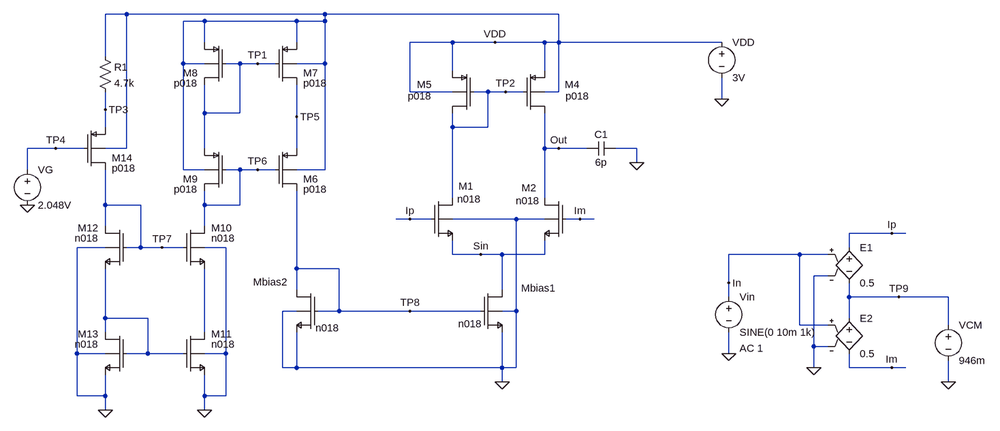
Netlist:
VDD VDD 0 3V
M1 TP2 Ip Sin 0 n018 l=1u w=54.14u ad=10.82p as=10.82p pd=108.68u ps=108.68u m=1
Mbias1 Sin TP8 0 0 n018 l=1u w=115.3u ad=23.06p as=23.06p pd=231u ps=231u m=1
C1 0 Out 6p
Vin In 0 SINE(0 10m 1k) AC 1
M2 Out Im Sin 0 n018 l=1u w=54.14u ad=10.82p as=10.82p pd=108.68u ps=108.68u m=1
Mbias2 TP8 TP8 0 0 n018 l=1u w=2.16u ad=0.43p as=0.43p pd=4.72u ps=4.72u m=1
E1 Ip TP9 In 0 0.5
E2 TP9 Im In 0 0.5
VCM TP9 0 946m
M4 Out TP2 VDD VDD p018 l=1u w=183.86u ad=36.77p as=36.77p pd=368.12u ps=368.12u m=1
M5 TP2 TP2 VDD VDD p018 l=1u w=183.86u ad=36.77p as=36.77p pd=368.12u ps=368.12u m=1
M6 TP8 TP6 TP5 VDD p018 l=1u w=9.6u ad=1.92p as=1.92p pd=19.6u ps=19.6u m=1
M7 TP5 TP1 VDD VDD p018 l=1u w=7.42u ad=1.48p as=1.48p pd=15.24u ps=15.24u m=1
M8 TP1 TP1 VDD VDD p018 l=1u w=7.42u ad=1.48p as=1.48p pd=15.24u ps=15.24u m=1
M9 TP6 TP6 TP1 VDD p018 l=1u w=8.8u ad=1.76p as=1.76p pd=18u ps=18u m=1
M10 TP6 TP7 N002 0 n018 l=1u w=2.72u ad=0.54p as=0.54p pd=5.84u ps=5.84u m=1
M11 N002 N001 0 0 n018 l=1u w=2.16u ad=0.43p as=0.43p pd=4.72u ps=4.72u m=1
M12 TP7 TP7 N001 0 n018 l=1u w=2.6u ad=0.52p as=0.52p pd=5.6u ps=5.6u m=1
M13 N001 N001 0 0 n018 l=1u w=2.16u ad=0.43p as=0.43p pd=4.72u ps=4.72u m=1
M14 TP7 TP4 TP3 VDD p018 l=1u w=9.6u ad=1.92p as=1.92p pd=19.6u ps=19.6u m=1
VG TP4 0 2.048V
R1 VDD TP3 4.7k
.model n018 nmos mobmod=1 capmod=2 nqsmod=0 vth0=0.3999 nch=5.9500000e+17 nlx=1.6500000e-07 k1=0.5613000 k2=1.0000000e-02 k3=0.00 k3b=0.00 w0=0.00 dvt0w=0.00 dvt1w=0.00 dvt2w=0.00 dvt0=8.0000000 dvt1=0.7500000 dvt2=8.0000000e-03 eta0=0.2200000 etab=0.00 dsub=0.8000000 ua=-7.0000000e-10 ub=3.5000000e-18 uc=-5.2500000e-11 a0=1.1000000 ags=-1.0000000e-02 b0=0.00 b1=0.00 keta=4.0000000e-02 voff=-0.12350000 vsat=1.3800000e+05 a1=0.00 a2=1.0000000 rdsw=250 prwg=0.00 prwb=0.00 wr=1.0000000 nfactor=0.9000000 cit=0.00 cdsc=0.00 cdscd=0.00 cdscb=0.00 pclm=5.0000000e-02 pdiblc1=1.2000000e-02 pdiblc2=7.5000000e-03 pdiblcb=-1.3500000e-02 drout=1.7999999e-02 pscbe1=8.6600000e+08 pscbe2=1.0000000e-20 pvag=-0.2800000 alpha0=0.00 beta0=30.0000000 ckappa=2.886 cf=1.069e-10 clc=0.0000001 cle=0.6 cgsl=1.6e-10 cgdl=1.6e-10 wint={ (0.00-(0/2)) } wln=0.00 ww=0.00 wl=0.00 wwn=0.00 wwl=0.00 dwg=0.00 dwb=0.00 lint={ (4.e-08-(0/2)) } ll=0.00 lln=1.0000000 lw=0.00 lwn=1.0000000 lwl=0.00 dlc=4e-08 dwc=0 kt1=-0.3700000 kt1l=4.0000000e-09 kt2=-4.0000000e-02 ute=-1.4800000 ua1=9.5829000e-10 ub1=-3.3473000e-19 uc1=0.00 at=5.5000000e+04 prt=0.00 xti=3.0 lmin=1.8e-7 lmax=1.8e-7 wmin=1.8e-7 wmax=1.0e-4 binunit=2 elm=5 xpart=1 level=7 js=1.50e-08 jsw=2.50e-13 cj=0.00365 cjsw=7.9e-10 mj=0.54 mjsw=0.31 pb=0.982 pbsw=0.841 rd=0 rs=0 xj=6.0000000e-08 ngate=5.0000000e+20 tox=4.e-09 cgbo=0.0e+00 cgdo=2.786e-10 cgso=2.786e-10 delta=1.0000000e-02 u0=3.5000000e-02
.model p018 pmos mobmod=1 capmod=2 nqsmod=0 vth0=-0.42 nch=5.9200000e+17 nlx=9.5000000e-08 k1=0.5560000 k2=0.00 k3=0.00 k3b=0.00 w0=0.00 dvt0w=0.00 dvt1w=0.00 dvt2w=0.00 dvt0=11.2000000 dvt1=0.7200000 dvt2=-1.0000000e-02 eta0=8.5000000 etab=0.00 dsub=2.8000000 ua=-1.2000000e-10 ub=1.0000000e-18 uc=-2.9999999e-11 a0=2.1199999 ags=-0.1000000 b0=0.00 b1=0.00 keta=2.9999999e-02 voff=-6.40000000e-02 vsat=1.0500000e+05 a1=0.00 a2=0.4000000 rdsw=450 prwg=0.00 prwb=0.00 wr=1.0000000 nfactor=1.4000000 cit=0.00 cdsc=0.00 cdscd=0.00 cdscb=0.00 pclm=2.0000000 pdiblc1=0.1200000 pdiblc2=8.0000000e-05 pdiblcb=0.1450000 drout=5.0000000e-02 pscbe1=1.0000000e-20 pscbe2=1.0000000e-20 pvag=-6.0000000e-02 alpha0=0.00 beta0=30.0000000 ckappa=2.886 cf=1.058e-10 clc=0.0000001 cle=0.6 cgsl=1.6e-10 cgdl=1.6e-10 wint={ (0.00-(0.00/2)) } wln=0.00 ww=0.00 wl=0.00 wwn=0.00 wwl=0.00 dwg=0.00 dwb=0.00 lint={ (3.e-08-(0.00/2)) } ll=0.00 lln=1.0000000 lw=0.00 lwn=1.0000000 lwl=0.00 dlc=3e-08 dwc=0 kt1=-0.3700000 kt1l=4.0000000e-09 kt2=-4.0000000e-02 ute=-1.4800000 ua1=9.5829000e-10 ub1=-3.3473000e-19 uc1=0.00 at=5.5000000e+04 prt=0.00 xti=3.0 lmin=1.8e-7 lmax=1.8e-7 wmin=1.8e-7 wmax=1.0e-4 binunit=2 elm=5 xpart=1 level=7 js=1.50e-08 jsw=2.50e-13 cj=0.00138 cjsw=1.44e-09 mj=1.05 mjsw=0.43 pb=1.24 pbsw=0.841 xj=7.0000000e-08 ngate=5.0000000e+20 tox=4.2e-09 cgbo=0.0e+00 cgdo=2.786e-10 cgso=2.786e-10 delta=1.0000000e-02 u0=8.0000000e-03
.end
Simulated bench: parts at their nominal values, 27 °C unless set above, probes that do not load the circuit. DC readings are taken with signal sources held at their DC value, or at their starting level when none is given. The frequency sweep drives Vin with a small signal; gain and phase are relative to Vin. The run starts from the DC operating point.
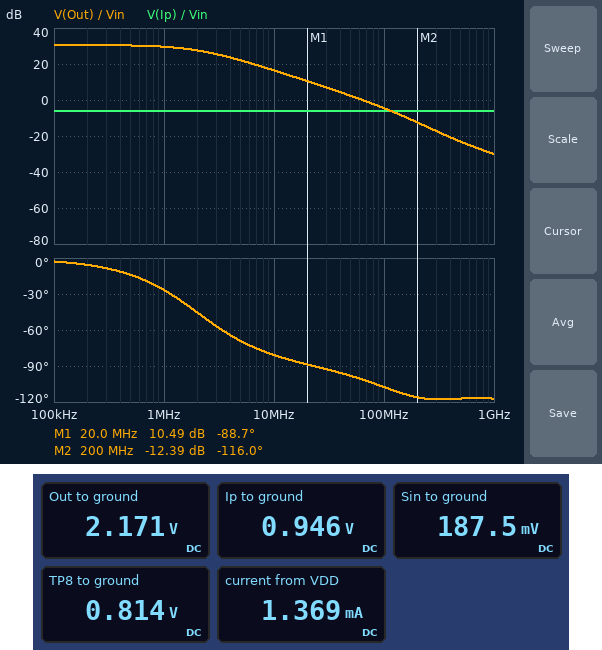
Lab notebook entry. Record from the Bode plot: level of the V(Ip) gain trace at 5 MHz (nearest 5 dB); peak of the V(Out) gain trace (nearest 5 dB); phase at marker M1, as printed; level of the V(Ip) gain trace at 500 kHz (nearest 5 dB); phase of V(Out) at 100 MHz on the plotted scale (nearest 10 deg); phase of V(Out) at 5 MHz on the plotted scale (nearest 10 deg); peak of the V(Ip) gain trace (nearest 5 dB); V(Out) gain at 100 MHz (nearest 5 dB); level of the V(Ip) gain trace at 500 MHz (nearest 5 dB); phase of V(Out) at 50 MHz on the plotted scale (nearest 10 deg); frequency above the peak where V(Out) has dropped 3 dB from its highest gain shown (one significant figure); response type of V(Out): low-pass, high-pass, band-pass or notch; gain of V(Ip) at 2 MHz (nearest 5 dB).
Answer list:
-5 dB
30 dB
-88.7 deg
-5 dB
-110 deg
-70 deg
-5 dB
-5 dB
-5 dB
-100 deg
2 MHz
low-pass
-5 dB
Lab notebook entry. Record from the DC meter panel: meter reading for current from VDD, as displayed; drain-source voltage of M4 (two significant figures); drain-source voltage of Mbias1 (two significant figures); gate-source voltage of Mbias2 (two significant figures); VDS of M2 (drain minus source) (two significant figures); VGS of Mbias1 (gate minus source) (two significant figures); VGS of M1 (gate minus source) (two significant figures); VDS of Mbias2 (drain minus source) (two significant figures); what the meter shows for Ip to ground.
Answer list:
1.369 mA
-830 mV
190 mV
810 mV
2.0 V
810 mV
760 mV
810 mV
0.946 V
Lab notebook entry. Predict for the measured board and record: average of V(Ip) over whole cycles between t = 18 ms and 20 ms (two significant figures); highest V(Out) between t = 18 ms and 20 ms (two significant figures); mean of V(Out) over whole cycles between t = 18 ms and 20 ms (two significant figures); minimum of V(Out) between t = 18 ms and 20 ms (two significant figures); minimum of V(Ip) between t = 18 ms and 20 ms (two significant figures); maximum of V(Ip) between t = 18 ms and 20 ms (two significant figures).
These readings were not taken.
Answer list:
950 mV
2.4 V
2.1 V
1.6 V
940 mV
950 mV
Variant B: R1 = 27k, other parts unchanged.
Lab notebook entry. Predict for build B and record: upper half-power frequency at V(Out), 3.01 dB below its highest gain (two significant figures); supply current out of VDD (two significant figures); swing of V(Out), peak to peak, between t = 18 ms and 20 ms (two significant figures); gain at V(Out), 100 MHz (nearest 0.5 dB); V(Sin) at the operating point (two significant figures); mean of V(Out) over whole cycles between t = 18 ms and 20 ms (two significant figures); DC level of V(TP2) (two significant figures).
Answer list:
1.6 MHz
820 µA
880 mV
-6.5 dB
270 mV
2.2 V
2.3 V
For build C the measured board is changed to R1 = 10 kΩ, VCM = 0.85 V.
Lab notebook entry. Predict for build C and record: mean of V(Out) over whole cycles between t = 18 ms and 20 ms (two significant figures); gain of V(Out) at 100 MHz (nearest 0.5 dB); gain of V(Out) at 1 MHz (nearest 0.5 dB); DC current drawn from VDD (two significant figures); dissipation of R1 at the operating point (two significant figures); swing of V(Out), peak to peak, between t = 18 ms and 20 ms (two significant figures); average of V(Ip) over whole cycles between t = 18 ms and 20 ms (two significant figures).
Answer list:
2.2 V
-5.5 dB
28.5 dB
1.0 mA
3.6 µW
680 mV
850 mV
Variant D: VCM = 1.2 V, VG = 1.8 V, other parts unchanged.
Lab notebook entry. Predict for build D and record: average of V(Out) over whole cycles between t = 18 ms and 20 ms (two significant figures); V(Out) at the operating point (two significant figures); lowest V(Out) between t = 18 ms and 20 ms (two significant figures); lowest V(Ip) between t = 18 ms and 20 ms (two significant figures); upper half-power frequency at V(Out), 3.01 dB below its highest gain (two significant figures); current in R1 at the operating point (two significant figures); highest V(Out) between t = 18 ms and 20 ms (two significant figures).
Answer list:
1.9 V
2.0 V
1.3 V
1.2 V
1.5 MHz
46 µA
2.3 V
